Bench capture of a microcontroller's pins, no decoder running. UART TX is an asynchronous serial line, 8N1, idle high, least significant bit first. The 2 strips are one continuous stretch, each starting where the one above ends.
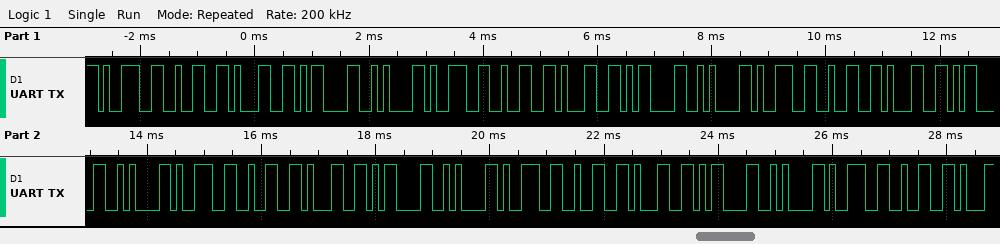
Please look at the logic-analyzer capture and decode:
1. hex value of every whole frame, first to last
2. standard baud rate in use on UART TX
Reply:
39 32 31 0D 0A 39 32 31 0D 0A 39 32 31 0D 0A 39 32 31 0D 0A 39 32 31 0D 0A 39 32
9600 baud
